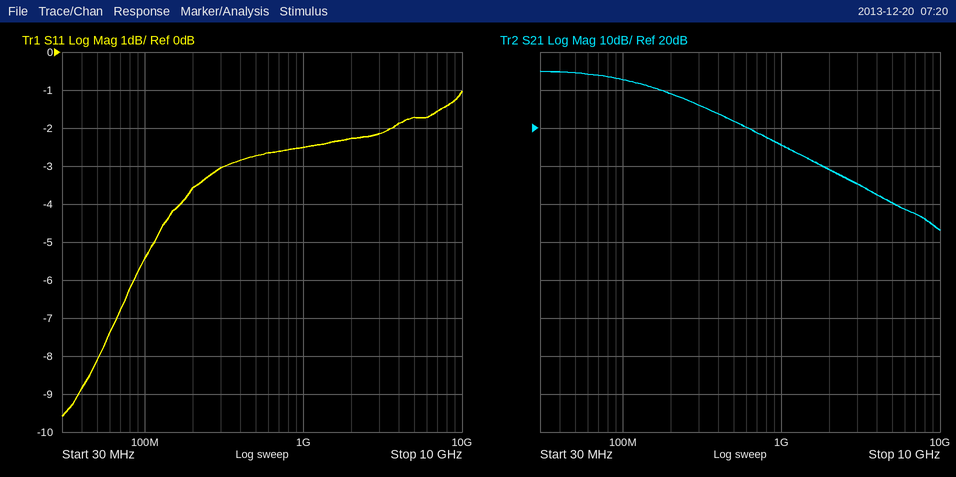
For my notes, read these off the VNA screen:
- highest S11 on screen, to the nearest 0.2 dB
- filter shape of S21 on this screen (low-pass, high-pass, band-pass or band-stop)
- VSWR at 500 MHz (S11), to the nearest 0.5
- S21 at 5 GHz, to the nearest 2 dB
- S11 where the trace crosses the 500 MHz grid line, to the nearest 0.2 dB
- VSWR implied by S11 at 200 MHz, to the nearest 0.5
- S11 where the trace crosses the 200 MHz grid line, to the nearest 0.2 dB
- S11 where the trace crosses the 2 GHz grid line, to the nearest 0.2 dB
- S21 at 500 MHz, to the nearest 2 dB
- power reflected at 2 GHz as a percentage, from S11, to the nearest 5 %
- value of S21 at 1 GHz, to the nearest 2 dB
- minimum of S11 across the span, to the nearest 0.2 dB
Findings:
-1.0 dB
low-pass
6.5
0 dB
-2.8 dB
5.0
-3.6 dB
-2.2 dB
22 dB
60 %
16 dB
-9.6 dB
